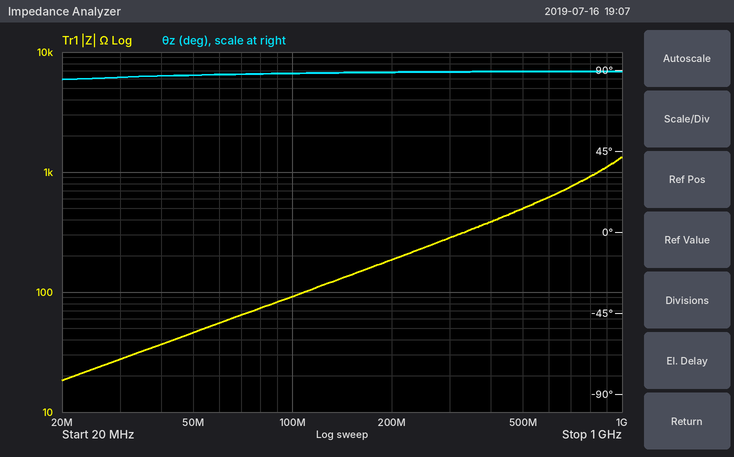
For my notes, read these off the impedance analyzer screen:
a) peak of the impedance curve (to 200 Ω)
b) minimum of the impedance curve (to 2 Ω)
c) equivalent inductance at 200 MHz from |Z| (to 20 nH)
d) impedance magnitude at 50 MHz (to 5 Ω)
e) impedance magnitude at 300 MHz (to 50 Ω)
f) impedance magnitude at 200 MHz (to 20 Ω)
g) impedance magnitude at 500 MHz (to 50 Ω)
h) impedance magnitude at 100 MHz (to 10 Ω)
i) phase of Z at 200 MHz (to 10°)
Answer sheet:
1.4 kΩ
18 Ω
140 nH
45 Ω
300 Ω
180 Ω
500 Ω
90 Ω
90°
